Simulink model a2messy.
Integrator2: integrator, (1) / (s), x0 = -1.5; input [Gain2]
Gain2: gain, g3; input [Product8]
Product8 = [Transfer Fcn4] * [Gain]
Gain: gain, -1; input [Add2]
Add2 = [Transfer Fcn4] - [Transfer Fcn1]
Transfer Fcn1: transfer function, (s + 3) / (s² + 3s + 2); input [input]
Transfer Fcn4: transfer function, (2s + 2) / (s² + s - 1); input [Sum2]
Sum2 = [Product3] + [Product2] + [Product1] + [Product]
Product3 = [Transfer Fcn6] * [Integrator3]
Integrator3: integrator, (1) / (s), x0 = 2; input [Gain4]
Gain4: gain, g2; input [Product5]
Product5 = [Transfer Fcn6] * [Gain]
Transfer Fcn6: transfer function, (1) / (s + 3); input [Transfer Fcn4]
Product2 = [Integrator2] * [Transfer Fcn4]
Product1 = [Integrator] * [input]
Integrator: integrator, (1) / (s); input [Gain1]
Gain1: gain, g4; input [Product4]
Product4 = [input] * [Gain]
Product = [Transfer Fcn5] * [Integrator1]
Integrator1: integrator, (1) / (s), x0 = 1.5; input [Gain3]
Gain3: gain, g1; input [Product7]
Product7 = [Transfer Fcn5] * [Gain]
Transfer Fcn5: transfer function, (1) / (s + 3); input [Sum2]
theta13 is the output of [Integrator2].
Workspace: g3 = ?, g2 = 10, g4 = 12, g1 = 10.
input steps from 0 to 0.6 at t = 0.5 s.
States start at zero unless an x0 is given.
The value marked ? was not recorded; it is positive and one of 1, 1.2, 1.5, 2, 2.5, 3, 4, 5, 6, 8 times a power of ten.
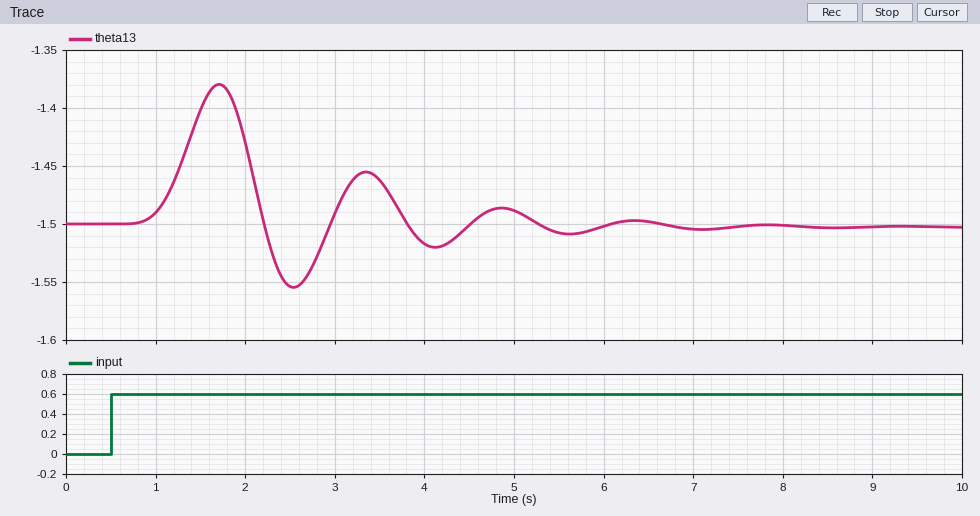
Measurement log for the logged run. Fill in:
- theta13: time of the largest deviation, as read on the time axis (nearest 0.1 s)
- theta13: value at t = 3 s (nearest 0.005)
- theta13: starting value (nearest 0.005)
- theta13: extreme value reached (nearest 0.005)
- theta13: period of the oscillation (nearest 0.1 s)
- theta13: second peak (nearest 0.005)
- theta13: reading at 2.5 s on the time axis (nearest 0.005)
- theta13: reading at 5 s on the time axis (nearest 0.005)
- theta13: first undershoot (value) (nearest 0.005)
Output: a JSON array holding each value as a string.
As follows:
["1.7 s", "-1.490", "-1.500", "-1.380", "1.6 s", "-1.455", "-1.555", "-1.490", "-1.555"]
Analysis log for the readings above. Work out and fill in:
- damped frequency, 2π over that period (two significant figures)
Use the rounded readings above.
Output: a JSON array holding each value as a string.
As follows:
["3.9 rad/s"]
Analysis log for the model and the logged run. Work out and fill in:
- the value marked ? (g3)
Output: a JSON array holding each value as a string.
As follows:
["5"]
